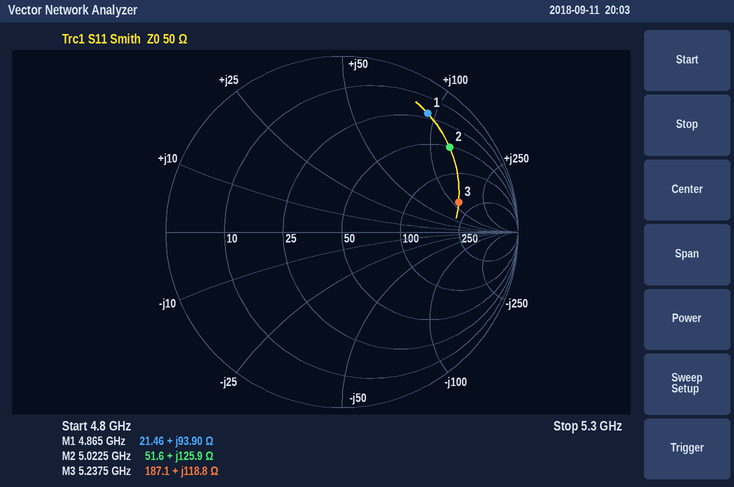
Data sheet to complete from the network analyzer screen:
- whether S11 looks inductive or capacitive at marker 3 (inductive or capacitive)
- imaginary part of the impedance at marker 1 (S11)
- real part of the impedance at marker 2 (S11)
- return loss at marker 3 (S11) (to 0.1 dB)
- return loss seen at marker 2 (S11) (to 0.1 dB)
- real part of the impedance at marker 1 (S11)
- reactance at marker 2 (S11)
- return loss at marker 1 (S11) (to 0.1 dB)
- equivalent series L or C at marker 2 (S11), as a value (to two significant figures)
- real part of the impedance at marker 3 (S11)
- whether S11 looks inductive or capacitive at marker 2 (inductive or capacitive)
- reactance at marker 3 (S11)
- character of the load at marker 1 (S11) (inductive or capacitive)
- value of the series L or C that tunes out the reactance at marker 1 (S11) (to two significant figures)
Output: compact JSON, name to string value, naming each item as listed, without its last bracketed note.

{"whether S11 looks inductive or capacitive at marker 3": "inductive", "imaginary part of the impedance at marker 1": "+93.90 Ω", "real part of the impedance at marker 2": "51.6 Ω", "return loss at marker 3 (S11)": "3.3 dB", "return loss seen at marker 2 (S11)": "2.2 dB", "real part of the impedance at marker 1": "21.46 Ω", "reactance at marker 2": "+125.9 Ω", "return loss at marker 1 (S11)": "1.6 dB", "equivalent series L or C at marker 2 (S11), as a value": "4.0 nH", "real part of the impedance at marker 3": "187.1 Ω", "whether S11 looks inductive or capacitive at marker 2": "inductive", "reactance at marker 3": "+118.8 Ω", "character of the load at marker 1 (S11)": "inductive", "value of the series L or C that tunes out the reactance at marker 1 (S11)": "350 fF"}
